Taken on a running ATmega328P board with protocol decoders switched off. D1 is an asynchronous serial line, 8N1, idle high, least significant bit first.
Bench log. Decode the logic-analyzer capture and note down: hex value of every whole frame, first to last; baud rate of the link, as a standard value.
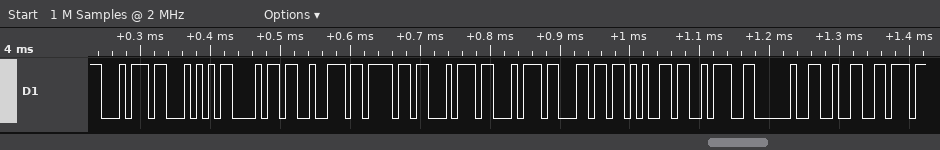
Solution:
0x74 0x54 0x68 0x72 0x6F 0x74 0x74 0x6C 0x65 0x3A 0x20 0x32
115200 baud
